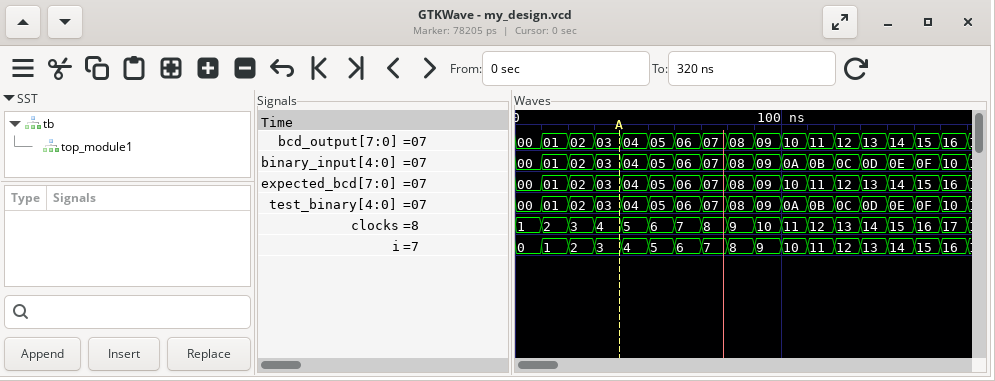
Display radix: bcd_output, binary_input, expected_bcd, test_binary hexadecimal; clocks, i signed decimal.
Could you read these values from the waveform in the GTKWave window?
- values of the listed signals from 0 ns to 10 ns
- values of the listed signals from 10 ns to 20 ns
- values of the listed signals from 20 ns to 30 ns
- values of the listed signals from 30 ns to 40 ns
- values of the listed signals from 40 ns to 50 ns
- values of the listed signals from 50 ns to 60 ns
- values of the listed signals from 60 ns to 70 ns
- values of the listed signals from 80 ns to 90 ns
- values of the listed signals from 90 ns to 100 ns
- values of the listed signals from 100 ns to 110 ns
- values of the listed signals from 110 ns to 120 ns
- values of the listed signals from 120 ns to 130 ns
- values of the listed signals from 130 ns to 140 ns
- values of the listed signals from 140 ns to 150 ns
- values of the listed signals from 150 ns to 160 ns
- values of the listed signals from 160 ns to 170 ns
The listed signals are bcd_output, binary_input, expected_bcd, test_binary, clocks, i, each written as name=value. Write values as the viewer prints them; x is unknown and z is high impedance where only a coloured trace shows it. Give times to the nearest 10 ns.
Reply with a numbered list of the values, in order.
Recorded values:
1. bcd_output=00, binary_input=00, expected_bcd=00, test_binary=00, clocks=1, i=0
2. bcd_output=01, binary_input=01, expected_bcd=01, test_binary=01, clocks=2, i=1
3. bcd_output=02, binary_input=02, expected_bcd=02, test_binary=02, clocks=3, i=2
4. bcd_output=03, binary_input=03, expected_bcd=03, test_binary=03, clocks=4, i=3
5. bcd_output=04, binary_input=04, expected_bcd=04, test_binary=04, clocks=5, i=4
6. bcd_output=05, binary_input=05, expected_bcd=05, test_binary=05, clocks=6, i=5
7. bcd_output=06, binary_input=06, expected_bcd=06, test_binary=06, clocks=7, i=6
8. bcd_output=08, binary_input=08, expected_bcd=08, test_binary=08, clocks=9, i=8
9. bcd_output=09, binary_input=09, expected_bcd=09, test_binary=09, clocks=10, i=9
10. bcd_output=10, binary_input=0A, expected_bcd=10, test_binary=0A, clocks=11, i=10
11. bcd_output=11, binary_input=0B, expected_bcd=11, test_binary=0B, clocks=12, i=11
12. bcd_output=12, binary_input=0C, expected_bcd=12, test_binary=0C, clocks=13, i=12
13. bcd_output=13, binary_input=0D, expected_bcd=13, test_binary=0D, clocks=14, i=13
14. bcd_output=14, binary_input=0E, expected_bcd=14, test_binary=0E, clocks=15, i=14
15. bcd_output=15, binary_input=0F, expected_bcd=15, test_binary=0F, clocks=16, i=15
16. bcd_output=16, binary_input=10, expected_bcd=16, test_binary=10, clocks=17, i=16
